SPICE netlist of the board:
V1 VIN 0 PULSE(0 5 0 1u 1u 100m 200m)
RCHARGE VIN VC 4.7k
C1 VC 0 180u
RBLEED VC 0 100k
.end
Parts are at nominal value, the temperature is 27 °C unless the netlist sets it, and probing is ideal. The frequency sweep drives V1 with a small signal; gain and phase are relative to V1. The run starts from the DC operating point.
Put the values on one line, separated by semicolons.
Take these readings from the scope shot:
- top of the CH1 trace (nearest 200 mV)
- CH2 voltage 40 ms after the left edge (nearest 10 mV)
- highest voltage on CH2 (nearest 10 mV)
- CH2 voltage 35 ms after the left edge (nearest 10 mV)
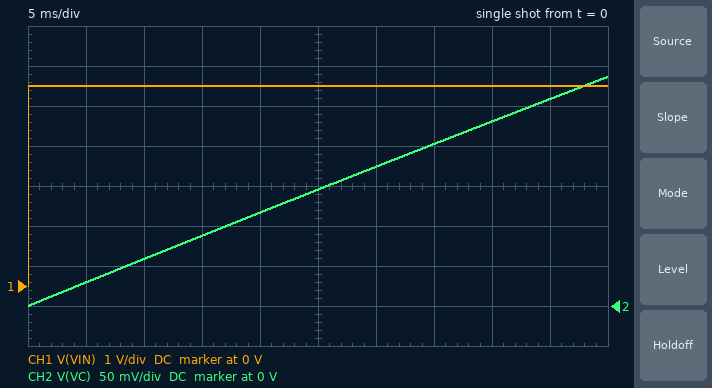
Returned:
5.0 V; 230 mV; 290 mV; 200 mV
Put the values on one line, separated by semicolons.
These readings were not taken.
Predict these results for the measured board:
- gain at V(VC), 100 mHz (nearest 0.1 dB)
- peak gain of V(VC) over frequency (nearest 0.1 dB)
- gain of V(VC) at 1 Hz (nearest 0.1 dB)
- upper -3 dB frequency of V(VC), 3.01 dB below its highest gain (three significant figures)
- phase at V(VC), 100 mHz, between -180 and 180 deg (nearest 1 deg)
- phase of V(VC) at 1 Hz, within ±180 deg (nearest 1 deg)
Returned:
-1.4 dB; -0.4 dB; -14.7 dB; 197 mHz; -27 deg; -79 deg
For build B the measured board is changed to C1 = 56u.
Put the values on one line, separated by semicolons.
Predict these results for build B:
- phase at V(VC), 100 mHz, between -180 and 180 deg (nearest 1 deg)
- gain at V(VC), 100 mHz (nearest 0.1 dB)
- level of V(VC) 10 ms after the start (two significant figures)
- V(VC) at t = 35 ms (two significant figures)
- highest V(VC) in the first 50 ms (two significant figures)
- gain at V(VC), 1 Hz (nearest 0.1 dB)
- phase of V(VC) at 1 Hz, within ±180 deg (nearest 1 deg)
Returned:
-9 deg; -0.5 dB; 190 mV; 620 mV; 860 mV; -5.8 dB; -58 deg
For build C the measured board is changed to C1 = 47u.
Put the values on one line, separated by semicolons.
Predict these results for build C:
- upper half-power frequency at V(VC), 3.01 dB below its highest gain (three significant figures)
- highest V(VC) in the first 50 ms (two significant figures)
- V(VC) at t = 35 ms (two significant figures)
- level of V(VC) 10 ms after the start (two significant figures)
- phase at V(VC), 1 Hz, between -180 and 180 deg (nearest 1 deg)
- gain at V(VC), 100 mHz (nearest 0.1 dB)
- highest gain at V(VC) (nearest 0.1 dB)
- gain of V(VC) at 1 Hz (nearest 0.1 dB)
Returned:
754 mHz; 1.0 V; 730 mV; 220 mV; -53 deg; -0.5 dB; -0.4 dB; -4.8 dB
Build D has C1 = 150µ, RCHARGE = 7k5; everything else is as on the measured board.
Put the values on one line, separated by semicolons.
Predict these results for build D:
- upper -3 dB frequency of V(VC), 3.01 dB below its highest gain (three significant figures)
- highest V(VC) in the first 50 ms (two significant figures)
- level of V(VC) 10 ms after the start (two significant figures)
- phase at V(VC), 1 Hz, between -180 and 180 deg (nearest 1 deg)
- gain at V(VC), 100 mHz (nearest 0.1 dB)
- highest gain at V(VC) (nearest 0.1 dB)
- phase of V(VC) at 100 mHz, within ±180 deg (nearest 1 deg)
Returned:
152 mHz; 220 mV; 44 mV; -81 deg; -2.2 dB; -0.6 dB; -33 deg
